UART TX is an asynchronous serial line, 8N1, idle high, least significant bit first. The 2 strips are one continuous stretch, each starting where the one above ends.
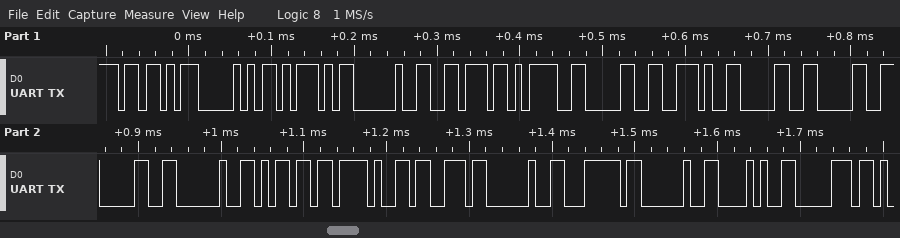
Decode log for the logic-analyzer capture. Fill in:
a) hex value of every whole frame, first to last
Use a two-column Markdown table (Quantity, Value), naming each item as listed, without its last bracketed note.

| Quantity | Value |
|---|---|
| hex value of every whole frame, first to last | 0x5B 0x50 0x5D 0x20 0x76 0x3D 0x30 0x2E 0x30 0x30 0x30 0x20 0x6D 0x2F 0x73 0x20 0x7C 0x20 0x28 0x70 |
